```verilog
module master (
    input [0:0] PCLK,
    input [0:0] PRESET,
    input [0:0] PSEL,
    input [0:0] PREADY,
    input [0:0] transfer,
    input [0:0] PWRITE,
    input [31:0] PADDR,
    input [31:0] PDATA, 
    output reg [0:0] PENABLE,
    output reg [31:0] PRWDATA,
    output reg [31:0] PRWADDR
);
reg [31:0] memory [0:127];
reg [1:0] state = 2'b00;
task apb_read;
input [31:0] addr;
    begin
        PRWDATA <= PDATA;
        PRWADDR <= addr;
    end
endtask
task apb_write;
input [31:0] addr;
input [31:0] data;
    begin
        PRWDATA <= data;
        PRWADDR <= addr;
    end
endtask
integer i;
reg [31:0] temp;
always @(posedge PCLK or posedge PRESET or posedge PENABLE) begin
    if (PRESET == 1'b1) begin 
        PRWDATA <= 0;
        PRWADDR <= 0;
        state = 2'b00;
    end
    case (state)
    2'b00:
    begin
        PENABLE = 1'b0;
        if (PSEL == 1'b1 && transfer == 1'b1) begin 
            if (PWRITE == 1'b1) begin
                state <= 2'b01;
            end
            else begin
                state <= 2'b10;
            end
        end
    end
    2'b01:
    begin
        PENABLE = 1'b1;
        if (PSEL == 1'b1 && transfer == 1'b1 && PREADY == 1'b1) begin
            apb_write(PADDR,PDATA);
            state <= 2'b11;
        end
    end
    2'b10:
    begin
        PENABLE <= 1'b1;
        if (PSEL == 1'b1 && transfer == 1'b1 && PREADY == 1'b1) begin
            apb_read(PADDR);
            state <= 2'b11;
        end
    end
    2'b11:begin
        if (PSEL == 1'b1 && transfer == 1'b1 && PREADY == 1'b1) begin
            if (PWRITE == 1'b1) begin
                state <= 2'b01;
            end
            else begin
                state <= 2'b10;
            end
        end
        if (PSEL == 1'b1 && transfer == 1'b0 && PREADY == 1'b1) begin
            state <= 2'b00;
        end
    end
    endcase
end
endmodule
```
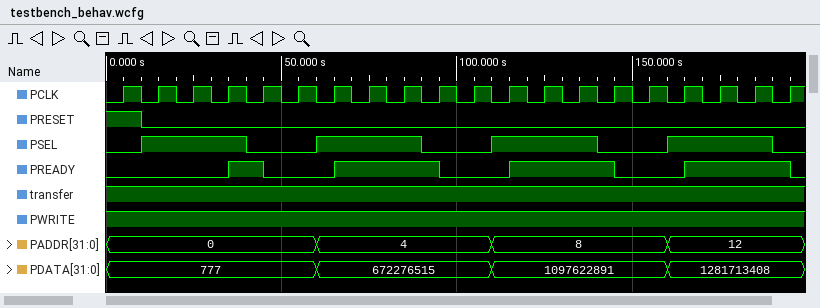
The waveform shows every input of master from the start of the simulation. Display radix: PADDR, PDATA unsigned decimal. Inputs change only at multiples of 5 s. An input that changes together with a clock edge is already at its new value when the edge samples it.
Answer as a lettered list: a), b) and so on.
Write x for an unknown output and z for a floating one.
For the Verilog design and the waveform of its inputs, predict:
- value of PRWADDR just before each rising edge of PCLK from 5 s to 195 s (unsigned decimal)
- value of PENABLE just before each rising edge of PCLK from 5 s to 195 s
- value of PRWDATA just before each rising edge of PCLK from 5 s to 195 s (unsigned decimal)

a) 0, 0, 0, 0, 0, 0, 0, 0, 4, 4, 4, 4, 8, 8, 8, 8, 8, 8, 12, 12
b) 0 0 0 1 1 1 1 1 1 1 1 1 1 1 1 1 1 1 1 1
c) 0, 0, 0, 0, 777, 777, 777, 777, 672276515, 672276515, 672276515, 672276515, 1097622891, 1097622891, 1097622891, 1097622891, 1097622891, 1097622891, 1281713408, 1281713408
